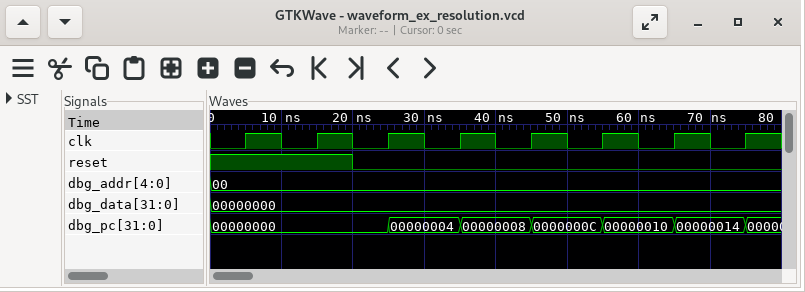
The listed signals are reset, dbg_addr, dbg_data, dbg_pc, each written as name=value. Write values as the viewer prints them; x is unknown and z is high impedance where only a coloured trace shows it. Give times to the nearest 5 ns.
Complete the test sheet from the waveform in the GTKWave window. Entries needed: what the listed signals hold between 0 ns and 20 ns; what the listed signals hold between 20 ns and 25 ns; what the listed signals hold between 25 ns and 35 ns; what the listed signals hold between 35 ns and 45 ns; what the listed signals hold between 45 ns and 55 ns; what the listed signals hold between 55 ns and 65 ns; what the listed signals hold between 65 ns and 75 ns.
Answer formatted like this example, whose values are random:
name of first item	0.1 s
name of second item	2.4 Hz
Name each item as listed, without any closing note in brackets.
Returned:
what the listed signals hold between 0 ns and 20 ns	reset=1, dbg_addr=00, dbg_data=00000000, dbg_pc=00000000
what the listed signals hold between 20 ns and 25 ns	reset=0, dbg_addr=00, dbg_data=00000000, dbg_pc=00000000
what the listed signals hold between 25 ns and 35 ns	reset=0, dbg_addr=00, dbg_data=00000000, dbg_pc=00000004
what the listed signals hold between 35 ns and 45 ns	reset=0, dbg_addr=00, dbg_data=00000000, dbg_pc=00000008
what the listed signals hold between 45 ns and 55 ns	reset=0, dbg_addr=00, dbg_data=00000000, dbg_pc=0000000C
what the listed signals hold between 55 ns and 65 ns	reset=0, dbg_addr=00, dbg_data=00000000, dbg_pc=00000010
what the listed signals hold between 65 ns and 75 ns	reset=0, dbg_addr=00, dbg_data=00000000, dbg_pc=00000014
